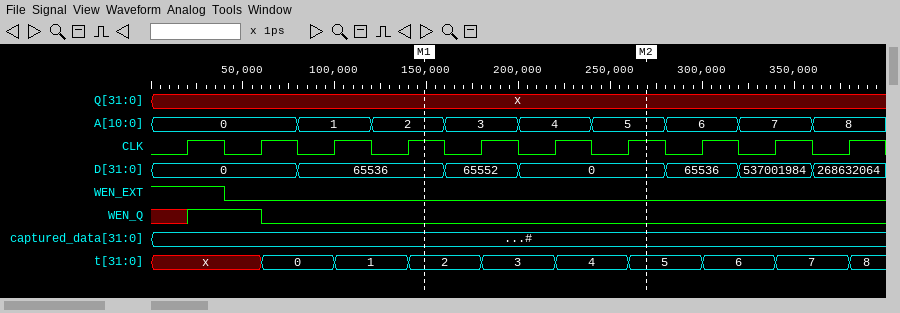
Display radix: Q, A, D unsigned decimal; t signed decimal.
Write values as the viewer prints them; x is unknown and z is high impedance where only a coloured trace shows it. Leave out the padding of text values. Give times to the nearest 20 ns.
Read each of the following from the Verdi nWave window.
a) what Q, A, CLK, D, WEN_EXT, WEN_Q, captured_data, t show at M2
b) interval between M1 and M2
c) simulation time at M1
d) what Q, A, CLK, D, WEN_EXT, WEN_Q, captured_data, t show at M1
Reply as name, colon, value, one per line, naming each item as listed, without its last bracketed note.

what Q, A, CLK, D, WEN_EXT, WEN_Q, captured_data, t show at M2: Q=x, A=5, CLK=1, D=0, WEN_EXT=0, WEN_Q=0, captured_data=#, t=5
interval between M1 and M2: 120 ns
simulation time at M1: 140 ns
what Q, A, CLK, D, WEN_EXT, WEN_Q, captured_data, t show at M1: Q=x, A=2, CLK=1, D=65536, WEN_EXT=0, WEN_Q=0, captured_data=#, t=2
